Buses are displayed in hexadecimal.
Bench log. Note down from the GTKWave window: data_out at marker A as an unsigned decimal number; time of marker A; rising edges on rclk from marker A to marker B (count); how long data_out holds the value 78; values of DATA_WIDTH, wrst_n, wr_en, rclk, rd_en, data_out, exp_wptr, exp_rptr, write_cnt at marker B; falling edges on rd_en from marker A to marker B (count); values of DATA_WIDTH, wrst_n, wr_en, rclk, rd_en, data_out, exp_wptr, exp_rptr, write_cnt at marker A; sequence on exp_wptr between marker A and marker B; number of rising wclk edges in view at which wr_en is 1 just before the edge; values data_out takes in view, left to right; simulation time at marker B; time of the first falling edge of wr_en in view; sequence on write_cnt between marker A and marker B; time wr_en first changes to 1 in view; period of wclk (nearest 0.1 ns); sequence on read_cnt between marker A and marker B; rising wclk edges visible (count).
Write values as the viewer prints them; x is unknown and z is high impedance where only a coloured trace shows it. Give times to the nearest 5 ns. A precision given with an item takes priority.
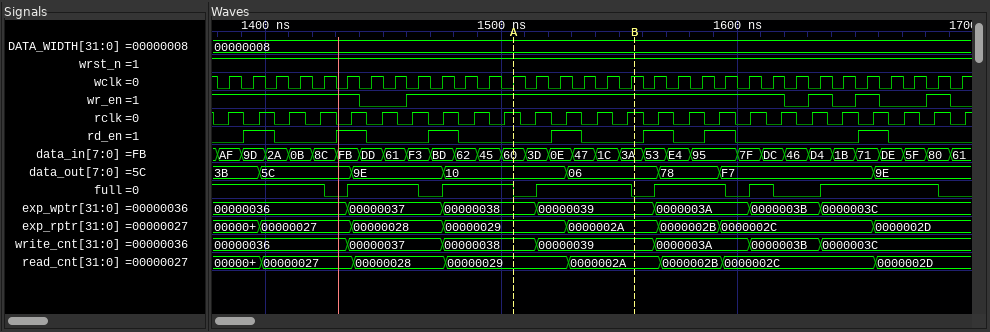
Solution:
16
1505 ns
4
25 ns
DATA_WIDTH=00000008, wrst_n=1, wr_en=1, rclk=1, rd_en=0, data_out=06, exp_wptr=00000039, exp_rptr=0000002A, write_cnt=00000039
1
DATA_WIDTH=00000008, wrst_n=1, wr_en=1, rclk=1, rd_en=0, data_out=10, exp_wptr=00000038, exp_rptr=00000029, write_cnt=00000038
00000038, 00000039
25
3B, 5C, 9E, 10, 06, 78, F7, 9E
1555 ns
1440 ns
00000038, 00000039
1460 ns
10 ns
00000029, 0000002A
32
